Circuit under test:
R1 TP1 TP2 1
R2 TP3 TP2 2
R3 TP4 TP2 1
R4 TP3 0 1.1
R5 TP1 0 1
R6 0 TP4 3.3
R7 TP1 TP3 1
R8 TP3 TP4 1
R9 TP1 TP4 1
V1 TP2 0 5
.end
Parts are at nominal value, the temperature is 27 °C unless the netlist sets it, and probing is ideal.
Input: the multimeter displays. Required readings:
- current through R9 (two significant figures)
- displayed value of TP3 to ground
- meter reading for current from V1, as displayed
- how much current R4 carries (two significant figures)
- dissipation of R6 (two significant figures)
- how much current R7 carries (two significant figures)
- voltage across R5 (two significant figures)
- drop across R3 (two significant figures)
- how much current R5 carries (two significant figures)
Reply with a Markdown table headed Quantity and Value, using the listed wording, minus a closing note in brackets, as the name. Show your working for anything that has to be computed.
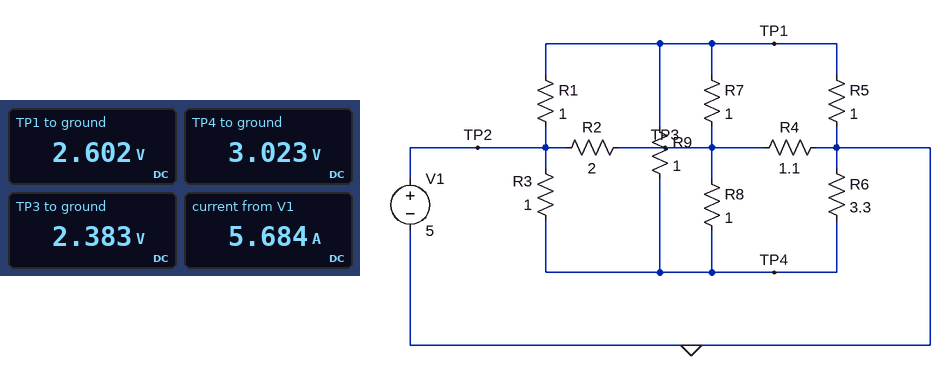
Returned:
| Quantity | Value |
|---|---|
| current through R9 | (3.023 V - 2.602 V) / 1 Ω = 420 mA |
| displayed value of TP3 to ground | 2.383 V |
| meter reading for current from V1, as displayed | 5.684 A |
| how much current R4 carries | (2.383 V) / 1.1 Ω = 2.2 A |
| dissipation of R6 | (3.023 V)^2 / 3.3 Ω = 2.8 W |
| how much current R7 carries | (2.602 V - 2.383 V) / 1 Ω = 220 mA |
| voltage across R5 | 2.602 V = 2.6 V |
| drop across R3 | 5 V - 3.023 V = 2.0 V |
| how much current R5 carries | (2.602 V) / 1 Ω = 2.6 A |
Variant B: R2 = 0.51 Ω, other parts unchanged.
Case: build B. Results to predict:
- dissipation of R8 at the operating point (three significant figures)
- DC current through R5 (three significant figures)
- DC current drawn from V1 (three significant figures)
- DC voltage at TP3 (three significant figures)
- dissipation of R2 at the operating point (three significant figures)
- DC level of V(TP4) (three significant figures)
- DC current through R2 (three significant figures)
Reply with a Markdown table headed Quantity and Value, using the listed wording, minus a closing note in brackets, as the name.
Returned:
| Quantity | Value |
|---|---|
| dissipation of R8 at the operating point | 8.13 mW |
| DC current through R5 | 2.93 A |
| DC current drawn from V1 | 6.97 A |
| DC voltage at TP3 | 3.31 V |
| dissipation of R2 at the operating point | 5.58 W |
| DC level of V(TP4) | 3.40 V |
| DC current through R2 | 3.31 A |
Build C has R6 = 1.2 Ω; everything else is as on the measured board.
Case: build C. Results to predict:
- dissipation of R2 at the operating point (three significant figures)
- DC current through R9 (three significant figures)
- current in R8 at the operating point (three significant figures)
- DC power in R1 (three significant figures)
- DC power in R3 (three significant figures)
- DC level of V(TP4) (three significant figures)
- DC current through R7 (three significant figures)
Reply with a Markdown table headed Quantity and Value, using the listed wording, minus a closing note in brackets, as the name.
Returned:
| Quantity | Value |
|---|---|
| dissipation of R2 at the operating point | 3.98 W |
| DC current through R9 | 83.5 mA |
| current in R8 at the operating point | 326 mA |
| DC power in R1 | 6.65 W |
| DC power in R3 | 6.23 W |
| DC level of V(TP4) | 2.50 V |
| DC current through R7 | 243 mA |
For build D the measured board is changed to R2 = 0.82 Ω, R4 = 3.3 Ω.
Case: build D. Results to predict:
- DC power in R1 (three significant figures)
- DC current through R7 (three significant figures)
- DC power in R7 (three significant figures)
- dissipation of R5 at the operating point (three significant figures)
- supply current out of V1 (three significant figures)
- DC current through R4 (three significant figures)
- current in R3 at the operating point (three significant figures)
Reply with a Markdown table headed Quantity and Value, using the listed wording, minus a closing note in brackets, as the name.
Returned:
| Quantity | Value |
|---|---|
| DC power in R1 | 3.90 W |
| DC current through R7 | 562 mA |
| DC power in R7 | 316 mW |
| dissipation of R5 at the operating point | 9.16 W |
| supply current out of V1 | 5.18 A |
| DC current through R4 | 1.09 A |
| current in R3 at the operating point | 1.48 A |
